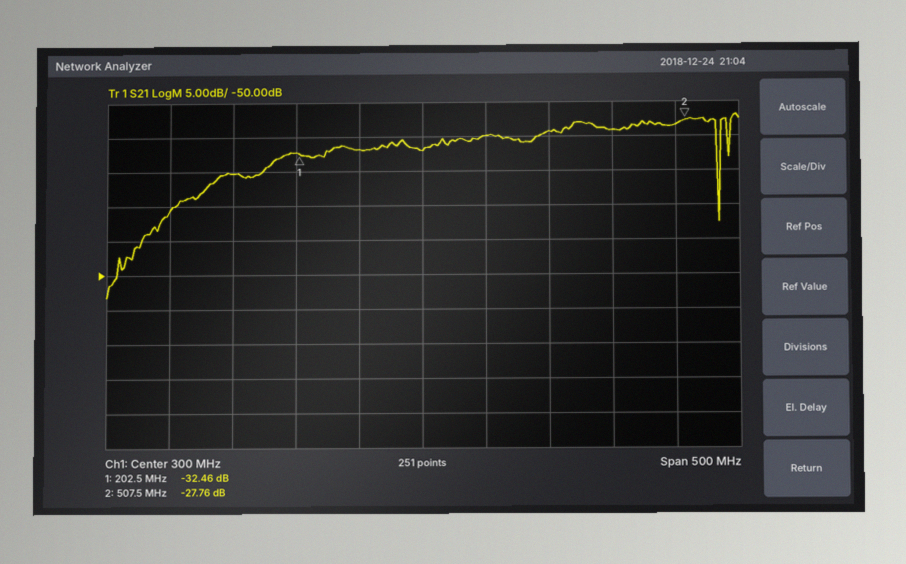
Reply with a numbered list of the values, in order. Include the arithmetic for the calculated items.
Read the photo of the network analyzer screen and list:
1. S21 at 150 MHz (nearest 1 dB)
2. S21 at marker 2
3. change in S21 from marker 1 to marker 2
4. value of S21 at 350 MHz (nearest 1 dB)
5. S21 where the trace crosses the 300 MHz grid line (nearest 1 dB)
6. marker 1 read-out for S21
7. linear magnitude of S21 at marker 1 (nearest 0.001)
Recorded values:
1. -35 dB
2. -27.76 dB
3. -27.76 − (-32.46) = 4.70 dB
4. -30 dB
5. -32 dB
6. -32.46 dB
7. 10^(-32.46/20) ≈ 0.024
